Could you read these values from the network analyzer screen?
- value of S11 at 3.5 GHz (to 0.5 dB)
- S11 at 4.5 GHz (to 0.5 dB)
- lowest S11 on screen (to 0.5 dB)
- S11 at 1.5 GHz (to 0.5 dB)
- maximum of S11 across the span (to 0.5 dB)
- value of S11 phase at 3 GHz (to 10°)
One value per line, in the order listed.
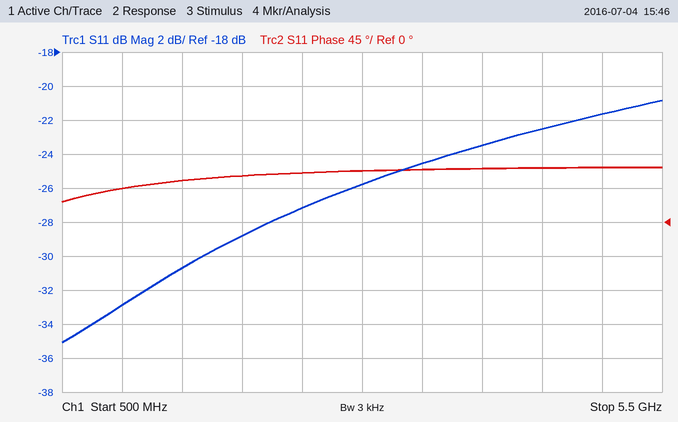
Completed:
-24.5 dB
-22.5 dB
-35.0 dB
-30.5 dB
-21.0 dB
70°
